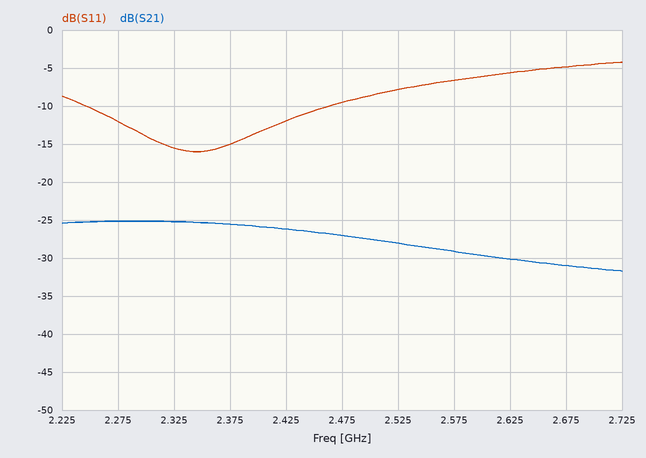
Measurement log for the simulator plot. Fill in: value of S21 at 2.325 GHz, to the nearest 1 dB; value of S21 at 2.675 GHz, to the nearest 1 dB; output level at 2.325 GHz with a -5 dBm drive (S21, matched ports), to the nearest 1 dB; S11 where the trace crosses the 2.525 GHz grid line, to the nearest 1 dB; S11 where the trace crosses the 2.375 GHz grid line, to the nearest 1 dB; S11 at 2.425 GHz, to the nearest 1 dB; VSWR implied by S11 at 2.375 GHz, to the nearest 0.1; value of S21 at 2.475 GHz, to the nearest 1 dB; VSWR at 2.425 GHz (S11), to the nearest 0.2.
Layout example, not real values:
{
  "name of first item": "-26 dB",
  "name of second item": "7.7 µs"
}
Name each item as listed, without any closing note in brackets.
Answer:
{
  "value of S21 at 2.325 GHz, to the nearest 1 dB": "-25 dB",
  "value of S21 at 2.675 GHz, to the nearest 1 dB": "-31 dB",
  "output level at 2.325 GHz with a -5 dBm drive (S21, matched ports), to the nearest 1 dB": "-30 dBm",
  "S11 where the trace crosses the 2.525 GHz grid line, to the nearest 1 dB": "-8 dB",
  "S11 where the trace crosses the 2.375 GHz grid line, to the nearest 1 dB": "-15 dB",
  "S11 at 2.425 GHz, to the nearest 1 dB": "-12 dB",
  "VSWR implied by S11 at 2.375 GHz, to the nearest 0.1": "1.4",
  "value of S21 at 2.475 GHz, to the nearest 1 dB": "-27 dB",
  "VSWR at 2.425 GHz (S11), to the nearest 0.2": "1.6"
}
